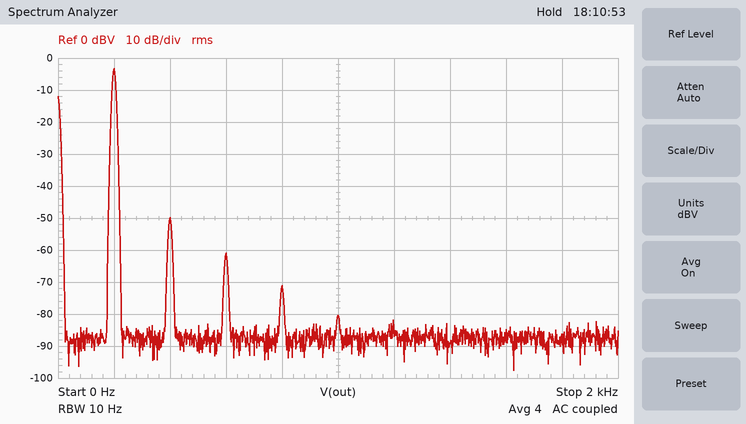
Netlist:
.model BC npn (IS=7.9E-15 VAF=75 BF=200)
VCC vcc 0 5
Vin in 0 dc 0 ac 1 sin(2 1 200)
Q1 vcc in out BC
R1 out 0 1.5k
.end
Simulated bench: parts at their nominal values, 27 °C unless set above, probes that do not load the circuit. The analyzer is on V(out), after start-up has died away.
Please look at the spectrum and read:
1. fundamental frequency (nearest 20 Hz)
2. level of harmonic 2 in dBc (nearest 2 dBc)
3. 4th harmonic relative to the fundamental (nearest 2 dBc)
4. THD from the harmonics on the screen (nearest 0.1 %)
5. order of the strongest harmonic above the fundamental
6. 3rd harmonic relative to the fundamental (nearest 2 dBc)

200 Hz
-46 dBc
-68 dBc
0.5 %
2
-58 dBc
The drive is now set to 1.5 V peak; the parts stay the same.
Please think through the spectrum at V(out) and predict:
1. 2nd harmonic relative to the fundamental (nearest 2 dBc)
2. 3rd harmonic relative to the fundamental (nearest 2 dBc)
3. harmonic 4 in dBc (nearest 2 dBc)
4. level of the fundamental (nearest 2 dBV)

-34 dBc
-38 dBc
-42 dBc
0 dBV
